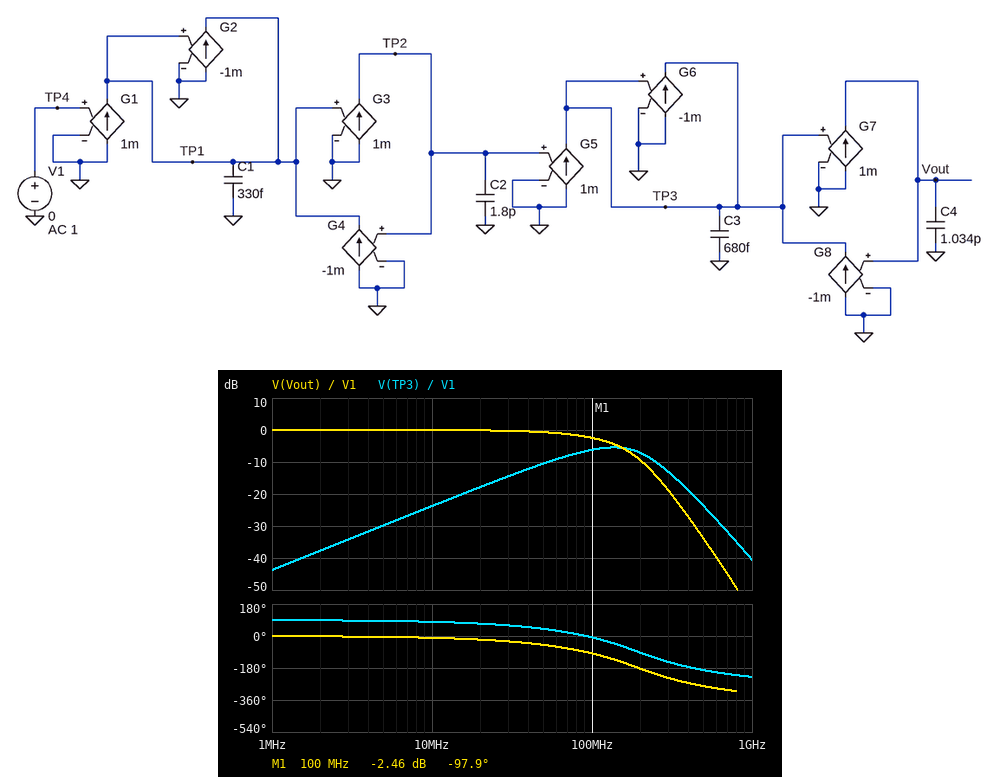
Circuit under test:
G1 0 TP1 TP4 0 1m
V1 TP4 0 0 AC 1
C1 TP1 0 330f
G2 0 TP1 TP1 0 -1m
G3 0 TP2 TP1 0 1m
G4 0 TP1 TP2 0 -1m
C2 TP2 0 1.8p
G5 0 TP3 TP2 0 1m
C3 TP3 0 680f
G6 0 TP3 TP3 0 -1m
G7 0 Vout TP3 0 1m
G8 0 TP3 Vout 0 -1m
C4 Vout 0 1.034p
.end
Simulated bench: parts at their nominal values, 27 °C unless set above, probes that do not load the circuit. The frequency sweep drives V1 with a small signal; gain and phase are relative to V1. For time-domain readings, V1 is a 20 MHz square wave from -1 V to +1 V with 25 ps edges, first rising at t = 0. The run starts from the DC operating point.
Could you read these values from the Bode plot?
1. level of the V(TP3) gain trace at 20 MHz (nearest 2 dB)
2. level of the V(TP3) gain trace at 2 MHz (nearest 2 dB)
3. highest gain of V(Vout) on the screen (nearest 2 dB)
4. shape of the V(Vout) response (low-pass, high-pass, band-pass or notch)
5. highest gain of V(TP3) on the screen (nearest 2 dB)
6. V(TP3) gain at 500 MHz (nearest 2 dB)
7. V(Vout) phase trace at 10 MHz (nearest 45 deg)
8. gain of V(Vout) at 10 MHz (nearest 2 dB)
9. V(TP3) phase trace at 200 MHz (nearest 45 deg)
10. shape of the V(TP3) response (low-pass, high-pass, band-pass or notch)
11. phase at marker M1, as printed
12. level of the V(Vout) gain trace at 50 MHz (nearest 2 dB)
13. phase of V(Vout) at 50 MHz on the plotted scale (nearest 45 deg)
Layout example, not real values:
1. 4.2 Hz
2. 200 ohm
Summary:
1. -18 dB
2. -38 dB
3. 0 dB
4. low-pass
5. -6 dB
6. -24 dB
7. 0 deg
8. 0 dB
9. -90 deg
10. band-pass
11. -97.9 deg
12. 0 dB
13. -45 deg
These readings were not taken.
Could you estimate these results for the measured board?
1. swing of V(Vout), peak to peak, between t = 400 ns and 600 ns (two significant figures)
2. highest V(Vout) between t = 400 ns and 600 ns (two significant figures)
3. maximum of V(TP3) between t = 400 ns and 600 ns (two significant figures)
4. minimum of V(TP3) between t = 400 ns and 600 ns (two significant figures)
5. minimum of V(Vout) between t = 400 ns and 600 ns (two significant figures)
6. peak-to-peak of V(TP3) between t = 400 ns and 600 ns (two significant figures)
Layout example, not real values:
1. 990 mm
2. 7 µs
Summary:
1. 2.0 V
2. 1.0 V
3. 690 mV
4. -690 mV
5. -1.0 V
6. 1.4 V
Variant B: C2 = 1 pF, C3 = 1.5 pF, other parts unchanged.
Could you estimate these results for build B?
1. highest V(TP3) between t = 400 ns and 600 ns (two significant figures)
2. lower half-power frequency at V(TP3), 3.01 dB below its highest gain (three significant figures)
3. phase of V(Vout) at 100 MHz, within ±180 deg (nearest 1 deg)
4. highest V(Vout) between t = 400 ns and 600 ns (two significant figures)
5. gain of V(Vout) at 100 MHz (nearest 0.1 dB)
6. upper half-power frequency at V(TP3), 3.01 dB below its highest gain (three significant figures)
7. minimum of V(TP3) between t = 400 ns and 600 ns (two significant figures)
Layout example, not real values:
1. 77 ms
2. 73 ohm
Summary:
1. 870 mV
2. 81.1 MHz
3. -95 deg
4. 1.4 V
5. 1.8 dB
6. 175 MHz
7. -870 mV
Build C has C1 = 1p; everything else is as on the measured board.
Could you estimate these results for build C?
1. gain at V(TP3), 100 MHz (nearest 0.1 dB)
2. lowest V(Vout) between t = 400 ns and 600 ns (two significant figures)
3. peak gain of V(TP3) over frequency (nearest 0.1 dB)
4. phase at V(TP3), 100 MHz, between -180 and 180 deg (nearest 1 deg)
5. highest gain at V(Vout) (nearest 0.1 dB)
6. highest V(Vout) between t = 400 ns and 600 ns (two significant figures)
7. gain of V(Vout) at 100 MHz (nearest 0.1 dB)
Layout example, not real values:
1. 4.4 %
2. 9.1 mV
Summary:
1. -4.8 dB
2. -1.2 V
3. -4.6 dB
4. -28 deg
5. 0.1 dB
6. 1.2 V
7. -1.1 dB
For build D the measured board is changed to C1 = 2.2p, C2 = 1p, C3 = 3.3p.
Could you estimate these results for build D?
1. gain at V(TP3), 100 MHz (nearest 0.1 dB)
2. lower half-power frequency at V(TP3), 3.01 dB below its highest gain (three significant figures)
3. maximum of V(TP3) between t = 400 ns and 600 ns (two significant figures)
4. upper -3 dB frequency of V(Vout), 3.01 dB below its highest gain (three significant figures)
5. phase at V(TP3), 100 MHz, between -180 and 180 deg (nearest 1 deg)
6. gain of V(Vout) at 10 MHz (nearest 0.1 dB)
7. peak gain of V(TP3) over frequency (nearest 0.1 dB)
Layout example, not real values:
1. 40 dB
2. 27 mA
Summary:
1. 2.8 dB
2. 69.7 MHz
3. 830 mV
4. 102 MHz
5. -106 deg
6. 0.2 dB
7. 3.8 dB
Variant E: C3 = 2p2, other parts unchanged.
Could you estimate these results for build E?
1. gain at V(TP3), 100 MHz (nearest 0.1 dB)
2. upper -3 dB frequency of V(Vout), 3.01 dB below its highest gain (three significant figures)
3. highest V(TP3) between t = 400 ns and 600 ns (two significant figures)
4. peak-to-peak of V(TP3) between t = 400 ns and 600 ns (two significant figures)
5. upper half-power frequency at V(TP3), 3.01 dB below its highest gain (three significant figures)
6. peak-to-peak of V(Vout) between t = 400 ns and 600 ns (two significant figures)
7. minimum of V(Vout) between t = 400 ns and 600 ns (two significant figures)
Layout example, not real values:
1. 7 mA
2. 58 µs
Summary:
1. -2.8 dB
2. 117 MHz
3. 660 mV
4. 1.3 V
5. 133 MHz
6. 2.8 V
7. -1.4 V
